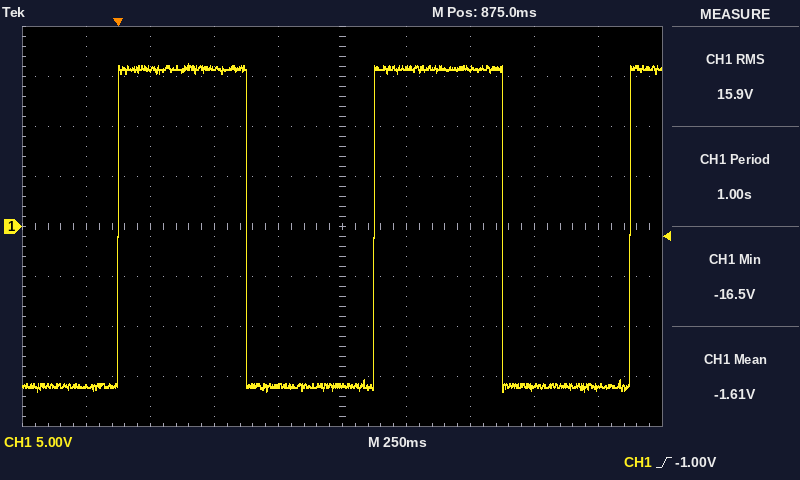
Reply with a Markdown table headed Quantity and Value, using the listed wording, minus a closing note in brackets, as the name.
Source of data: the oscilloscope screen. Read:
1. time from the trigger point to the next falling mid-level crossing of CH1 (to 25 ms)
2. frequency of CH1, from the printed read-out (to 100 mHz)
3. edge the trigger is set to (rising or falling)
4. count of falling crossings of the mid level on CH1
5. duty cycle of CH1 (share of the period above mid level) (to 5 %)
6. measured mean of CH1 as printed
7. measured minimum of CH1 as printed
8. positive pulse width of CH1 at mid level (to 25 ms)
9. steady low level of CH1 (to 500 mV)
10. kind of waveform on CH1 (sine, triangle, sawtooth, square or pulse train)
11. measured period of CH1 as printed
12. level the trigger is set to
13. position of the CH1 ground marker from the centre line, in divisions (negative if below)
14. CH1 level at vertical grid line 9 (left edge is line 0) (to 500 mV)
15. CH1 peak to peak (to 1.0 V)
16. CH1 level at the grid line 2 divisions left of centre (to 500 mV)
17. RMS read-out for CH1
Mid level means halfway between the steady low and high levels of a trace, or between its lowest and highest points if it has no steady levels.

| Quantity | Value |
|---|---|
| time from the trigger point to the next falling mid-level crossing of CH1 | 500 ms |
| frequency of CH1, from the printed read-out | 1.0 Hz |
| edge the trigger is set to | rising |
| count of falling crossings of the mid level on CH1 | 2 |
| duty cycle of CH1 (share of the period above mid level) | 50 % |
| measured mean of CH1 as printed | -1.61 V |
| measured minimum of CH1 as printed | -16.5 V |
| positive pulse width of CH1 at mid level | 500 ms |
| steady low level of CH1 | -16.0 V |
| kind of waveform on CH1 | square |
| measured period of CH1 as printed | 1.00 s |
| level the trigger is set to | -1.00 V |
| position of the CH1 ground marker from the centre line, in divisions | 0.0 div |
| CH1 level at vertical grid line 9 (left edge is line 0) | -16.0 V |
| CH1 peak to peak | 33.0 V |
| CH1 level at the grid line 2 divisions left of centre | 16.0 V |
| RMS read-out for CH1 | 15.9 V |
